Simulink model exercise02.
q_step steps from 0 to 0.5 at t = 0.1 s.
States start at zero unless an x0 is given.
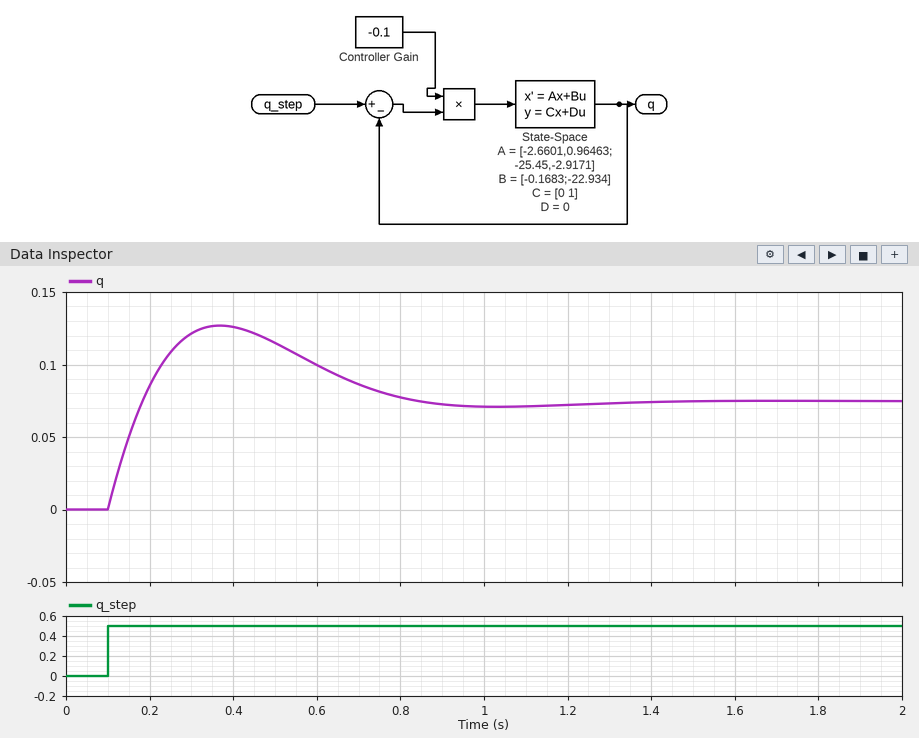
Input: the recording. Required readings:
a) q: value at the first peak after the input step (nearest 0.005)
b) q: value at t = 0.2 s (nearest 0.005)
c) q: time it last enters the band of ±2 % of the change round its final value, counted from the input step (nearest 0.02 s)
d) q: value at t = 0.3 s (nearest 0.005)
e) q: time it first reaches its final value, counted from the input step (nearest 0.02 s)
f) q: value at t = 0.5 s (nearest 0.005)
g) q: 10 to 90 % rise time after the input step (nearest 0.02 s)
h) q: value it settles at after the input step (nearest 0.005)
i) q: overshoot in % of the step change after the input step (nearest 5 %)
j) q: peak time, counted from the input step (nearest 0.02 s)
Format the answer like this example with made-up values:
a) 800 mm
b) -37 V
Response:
a) 0.125
b) 0.085
c) 1.20 s
d) 0.120
e) 0.08 s
f) 0.115
g) 0.06 s
h) 0.075
i) 70 %
j) 0.26 s
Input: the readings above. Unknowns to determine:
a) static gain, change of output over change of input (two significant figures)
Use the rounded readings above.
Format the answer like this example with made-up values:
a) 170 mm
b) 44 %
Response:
a) 0.15
